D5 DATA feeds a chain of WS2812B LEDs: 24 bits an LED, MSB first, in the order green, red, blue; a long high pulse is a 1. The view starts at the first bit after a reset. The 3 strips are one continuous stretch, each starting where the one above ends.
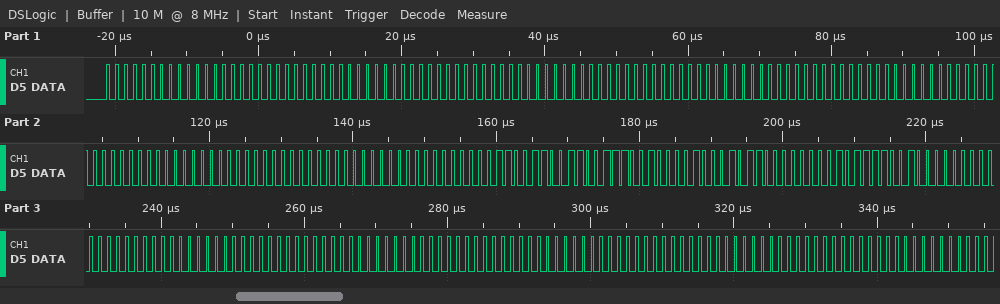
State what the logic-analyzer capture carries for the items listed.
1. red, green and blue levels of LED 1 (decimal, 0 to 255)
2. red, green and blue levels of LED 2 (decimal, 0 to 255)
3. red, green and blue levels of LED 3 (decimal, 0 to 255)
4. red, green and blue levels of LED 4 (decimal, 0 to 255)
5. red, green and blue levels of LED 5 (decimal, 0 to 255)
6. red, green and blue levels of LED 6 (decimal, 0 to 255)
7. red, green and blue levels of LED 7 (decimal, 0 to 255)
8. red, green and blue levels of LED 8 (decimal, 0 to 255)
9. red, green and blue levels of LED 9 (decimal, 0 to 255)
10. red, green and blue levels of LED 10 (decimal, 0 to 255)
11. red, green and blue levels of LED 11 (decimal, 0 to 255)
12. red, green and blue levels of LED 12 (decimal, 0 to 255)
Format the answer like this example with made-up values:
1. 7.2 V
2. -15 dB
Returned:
1. 0, 0, 0
2. 0, 0, 0
3. 0, 0, 0
4. 0, 0, 0
5. 0, 0, 0
6. 0, 0, 0
7. 103, 102, 33
8. 1, 22, 121
9. 0, 0, 0
10. 0, 0, 0
11. 0, 0, 0
12. 0, 0, 0
